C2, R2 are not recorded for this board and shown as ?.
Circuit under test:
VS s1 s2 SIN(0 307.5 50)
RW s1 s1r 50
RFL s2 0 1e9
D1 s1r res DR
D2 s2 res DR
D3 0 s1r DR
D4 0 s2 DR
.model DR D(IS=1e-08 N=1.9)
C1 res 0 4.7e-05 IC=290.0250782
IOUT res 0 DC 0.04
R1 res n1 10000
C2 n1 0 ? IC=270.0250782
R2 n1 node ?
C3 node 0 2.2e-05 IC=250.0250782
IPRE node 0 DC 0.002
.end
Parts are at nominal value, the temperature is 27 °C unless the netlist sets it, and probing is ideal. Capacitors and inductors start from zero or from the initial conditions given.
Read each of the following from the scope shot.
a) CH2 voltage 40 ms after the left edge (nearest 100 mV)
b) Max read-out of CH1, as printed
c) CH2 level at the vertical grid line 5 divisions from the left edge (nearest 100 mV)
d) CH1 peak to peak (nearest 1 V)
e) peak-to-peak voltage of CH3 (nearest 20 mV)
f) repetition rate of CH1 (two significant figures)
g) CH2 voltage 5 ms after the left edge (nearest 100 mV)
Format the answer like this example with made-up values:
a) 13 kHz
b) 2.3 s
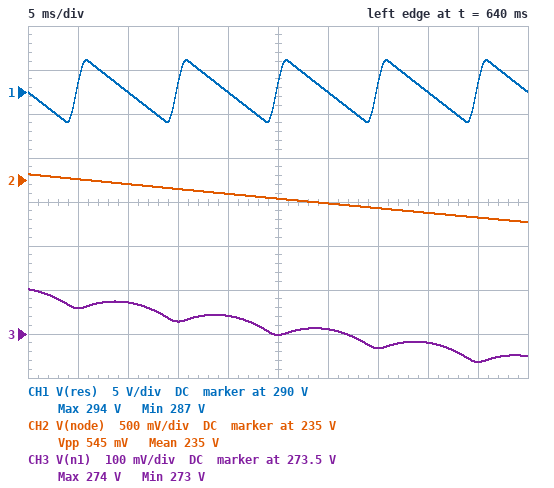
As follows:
a) 234.6 V
b) 294 V
c) 234.8 V
d) 7 V
e) 160 mV
f) 100 Hz
g) 235.0 V
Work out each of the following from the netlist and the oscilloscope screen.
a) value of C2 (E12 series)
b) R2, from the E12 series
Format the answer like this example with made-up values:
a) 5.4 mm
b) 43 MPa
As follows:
a) 33 µF
b) 22 kΩ
